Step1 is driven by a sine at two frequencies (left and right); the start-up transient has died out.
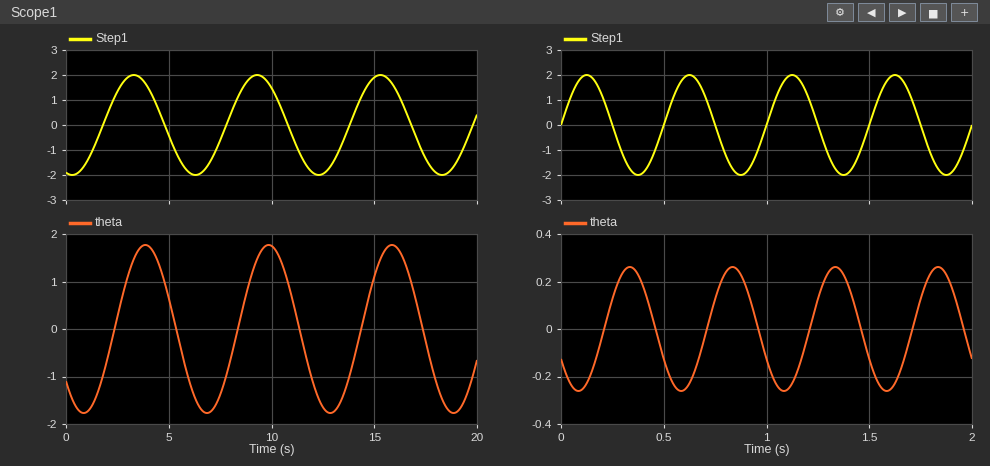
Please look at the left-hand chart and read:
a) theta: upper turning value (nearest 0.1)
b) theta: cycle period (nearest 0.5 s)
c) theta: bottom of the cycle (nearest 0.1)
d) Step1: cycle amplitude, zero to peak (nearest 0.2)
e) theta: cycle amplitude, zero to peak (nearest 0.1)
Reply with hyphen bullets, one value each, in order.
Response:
- 1.8
- 6.0 s
- -1.8
- 2.0
- 1.8
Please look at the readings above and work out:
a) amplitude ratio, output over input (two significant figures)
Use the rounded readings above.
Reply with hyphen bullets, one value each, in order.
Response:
- 0.90
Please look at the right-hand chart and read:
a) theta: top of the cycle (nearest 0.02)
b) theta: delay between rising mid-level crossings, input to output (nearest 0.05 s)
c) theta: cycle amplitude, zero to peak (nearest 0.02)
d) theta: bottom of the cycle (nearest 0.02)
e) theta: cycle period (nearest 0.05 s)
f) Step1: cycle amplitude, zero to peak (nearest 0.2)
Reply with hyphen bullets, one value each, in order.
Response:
- 0.26
- 0.20 s
- 0.26
- -0.26
- 0.50 s
- 2.0
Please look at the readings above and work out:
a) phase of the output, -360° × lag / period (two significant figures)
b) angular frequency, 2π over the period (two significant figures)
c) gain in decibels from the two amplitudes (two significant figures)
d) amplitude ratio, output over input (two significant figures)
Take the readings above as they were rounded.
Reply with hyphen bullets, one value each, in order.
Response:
- -140°
- 13 rad/s
- -18 dB
- 0.13
